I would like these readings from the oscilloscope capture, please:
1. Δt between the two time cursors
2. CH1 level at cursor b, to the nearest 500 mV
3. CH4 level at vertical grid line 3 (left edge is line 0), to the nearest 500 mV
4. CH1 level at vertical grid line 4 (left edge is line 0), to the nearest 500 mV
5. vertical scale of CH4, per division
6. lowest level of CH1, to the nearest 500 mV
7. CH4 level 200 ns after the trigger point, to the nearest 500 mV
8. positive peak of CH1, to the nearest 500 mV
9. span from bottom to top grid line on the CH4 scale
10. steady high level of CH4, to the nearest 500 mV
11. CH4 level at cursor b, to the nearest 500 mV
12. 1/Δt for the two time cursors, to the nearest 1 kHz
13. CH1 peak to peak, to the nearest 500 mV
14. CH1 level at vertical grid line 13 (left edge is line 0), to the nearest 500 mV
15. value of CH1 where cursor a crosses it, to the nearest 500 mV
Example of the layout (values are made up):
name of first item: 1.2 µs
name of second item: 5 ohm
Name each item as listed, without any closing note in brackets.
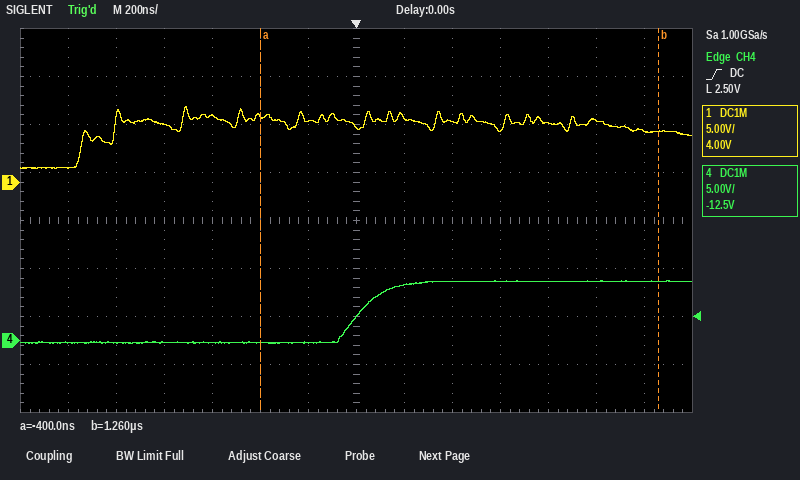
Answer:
Δt between the two time cursors: 1.66 µs
CH1 level at cursor b, to the nearest 500 mV: 5.5 V
CH4 level at vertical grid line 3 (left edge is line 0), to the nearest 500 mV: 0.0 V
CH1 level at vertical grid line 4 (left edge is line 0), to the nearest 500 mV: 7.0 V
vertical scale of CH4, per division: 5 V
lowest level of CH1, to the nearest 500 mV: 1.5 V
CH4 level 200 ns after the trigger point, to the nearest 500 mV: 6.0 V
positive peak of CH1, to the nearest 500 mV: 8.0 V
span from bottom to top grid line on the CH4 scale: 40 V
steady high level of CH4, to the nearest 500 mV: 6.0 V
CH4 level at cursor b, to the nearest 500 mV: 6.0 V
1/Δt for the two time cursors, to the nearest 1 kHz: 602 kHz
CH1 peak to peak, to the nearest 500 mV: 6.5 V
CH1 level at vertical grid line 13 (left edge is line 0), to the nearest 500 mV: 5.5 V
value of CH1 where cursor a crosses it, to the nearest 500 mV: 7.0 V
